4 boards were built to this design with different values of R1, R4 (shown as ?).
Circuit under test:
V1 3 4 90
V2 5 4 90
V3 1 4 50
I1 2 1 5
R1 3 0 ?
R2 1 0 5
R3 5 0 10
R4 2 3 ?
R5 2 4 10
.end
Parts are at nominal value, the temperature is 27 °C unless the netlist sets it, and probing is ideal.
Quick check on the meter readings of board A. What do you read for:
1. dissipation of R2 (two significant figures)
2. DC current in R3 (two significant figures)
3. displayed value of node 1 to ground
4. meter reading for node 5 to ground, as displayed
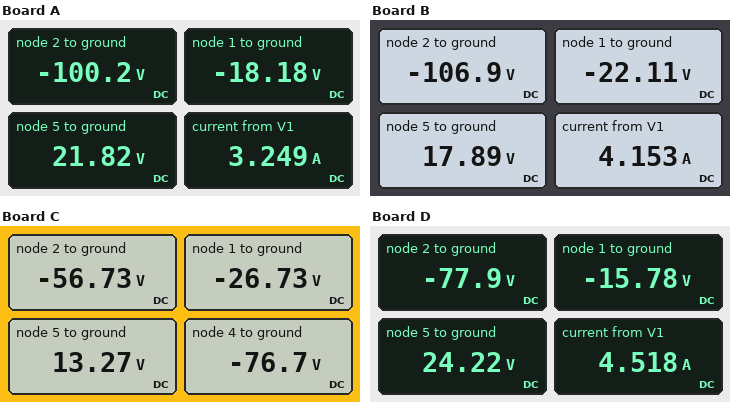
66 W
2.2 A
-18.18 V
21.82 V
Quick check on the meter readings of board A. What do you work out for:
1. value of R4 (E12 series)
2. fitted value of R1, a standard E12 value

68 Ω
15 Ω
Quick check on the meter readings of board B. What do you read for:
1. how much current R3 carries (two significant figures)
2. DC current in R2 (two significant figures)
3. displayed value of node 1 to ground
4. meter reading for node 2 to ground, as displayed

1.8 A
4.4 A
-22.11 V
-106.9 V
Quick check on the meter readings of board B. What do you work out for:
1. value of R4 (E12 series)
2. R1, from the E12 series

82 Ω
6.8 Ω
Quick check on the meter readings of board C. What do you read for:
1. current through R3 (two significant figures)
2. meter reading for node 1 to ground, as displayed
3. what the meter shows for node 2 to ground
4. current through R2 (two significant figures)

1.3 A
-26.73 V
-56.73 V
5.3 A
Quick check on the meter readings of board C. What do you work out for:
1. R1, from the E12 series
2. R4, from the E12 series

3.3 Ω
10 Ω
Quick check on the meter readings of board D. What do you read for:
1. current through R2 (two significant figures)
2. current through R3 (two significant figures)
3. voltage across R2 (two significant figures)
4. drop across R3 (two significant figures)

3.2 A
2.4 A
16 V
24 V
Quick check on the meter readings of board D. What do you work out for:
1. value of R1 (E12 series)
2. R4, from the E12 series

33 Ω
27 Ω
